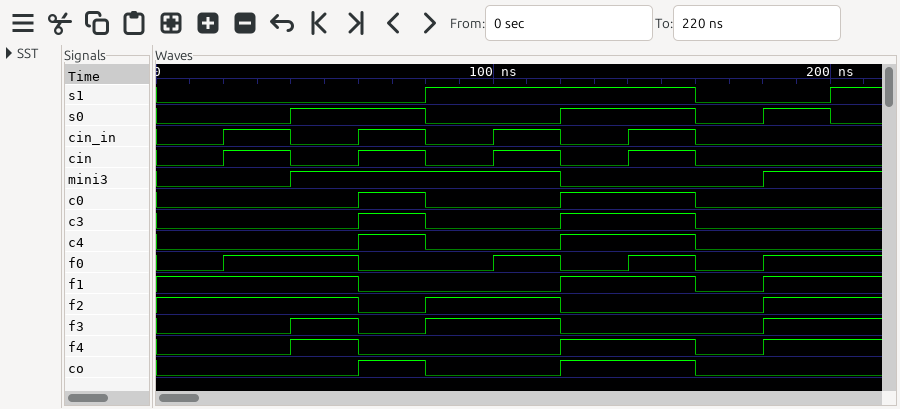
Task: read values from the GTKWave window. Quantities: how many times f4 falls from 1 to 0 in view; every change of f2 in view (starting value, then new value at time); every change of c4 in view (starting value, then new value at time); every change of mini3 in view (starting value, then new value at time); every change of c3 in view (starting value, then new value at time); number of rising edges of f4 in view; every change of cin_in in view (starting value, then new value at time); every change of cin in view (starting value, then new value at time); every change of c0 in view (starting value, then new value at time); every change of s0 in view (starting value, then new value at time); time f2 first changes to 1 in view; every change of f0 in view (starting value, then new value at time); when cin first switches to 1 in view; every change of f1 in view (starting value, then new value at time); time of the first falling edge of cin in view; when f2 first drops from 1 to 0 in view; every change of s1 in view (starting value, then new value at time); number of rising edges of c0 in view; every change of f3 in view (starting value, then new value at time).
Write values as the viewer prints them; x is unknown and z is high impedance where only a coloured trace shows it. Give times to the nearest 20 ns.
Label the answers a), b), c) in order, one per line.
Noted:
a) 2
b) 1, 0 at 60 ns, 1 at 80 ns, 0 at 120 ns, 1 at 180 ns
c) 0, 1 at 60 ns, 0 at 80 ns, 1 at 120 ns, 0 at 160 ns
d) 0, 1 at 40 ns, 0 at 120 ns, 1 at 180 ns
e) 0, 1 at 60 ns, 0 at 80 ns, 1 at 120 ns, 0 at 160 ns
f) 3
g) 0, 1 at 20 ns, 0 at 40 ns, 1 at 60 ns, 0 at 80 ns, 1 at 100 ns, 0 at 120 ns, 1 at 140 ns, 0 at 160 ns
h) 0, 1 at 20 ns, 0 at 40 ns, 1 at 60 ns, 0 at 80 ns, 1 at 100 ns, 0 at 120 ns, 1 at 140 ns, 0 at 160 ns
i) 0, 1 at 60 ns, 0 at 80 ns, 1 at 120 ns, 0 at 160 ns
j) 0, 1 at 40 ns, 0 at 80 ns, 1 at 120 ns, 0 at 160 ns, 1 at 180 ns, 0 at 200 ns
k) 80 ns
l) 0, 1 at 20 ns, 0 at 60 ns, 1 at 100 ns, 0 at 120 ns, 1 at 140 ns, 0 at 160 ns, 1 at 180 ns
m) 20 ns
n) 1, 0 at 60 ns, 1 at 120 ns, 0 at 160 ns, 1 at 180 ns
o) 40 ns
p) 60 ns
q) 0, 1 at 80 ns, 0 at 160 ns, 1 at 200 ns
r) 2
s) 0, 1 at 40 ns, 0 at 60 ns, 1 at 80 ns, 0 at 120 ns, 1 at 180 ns
